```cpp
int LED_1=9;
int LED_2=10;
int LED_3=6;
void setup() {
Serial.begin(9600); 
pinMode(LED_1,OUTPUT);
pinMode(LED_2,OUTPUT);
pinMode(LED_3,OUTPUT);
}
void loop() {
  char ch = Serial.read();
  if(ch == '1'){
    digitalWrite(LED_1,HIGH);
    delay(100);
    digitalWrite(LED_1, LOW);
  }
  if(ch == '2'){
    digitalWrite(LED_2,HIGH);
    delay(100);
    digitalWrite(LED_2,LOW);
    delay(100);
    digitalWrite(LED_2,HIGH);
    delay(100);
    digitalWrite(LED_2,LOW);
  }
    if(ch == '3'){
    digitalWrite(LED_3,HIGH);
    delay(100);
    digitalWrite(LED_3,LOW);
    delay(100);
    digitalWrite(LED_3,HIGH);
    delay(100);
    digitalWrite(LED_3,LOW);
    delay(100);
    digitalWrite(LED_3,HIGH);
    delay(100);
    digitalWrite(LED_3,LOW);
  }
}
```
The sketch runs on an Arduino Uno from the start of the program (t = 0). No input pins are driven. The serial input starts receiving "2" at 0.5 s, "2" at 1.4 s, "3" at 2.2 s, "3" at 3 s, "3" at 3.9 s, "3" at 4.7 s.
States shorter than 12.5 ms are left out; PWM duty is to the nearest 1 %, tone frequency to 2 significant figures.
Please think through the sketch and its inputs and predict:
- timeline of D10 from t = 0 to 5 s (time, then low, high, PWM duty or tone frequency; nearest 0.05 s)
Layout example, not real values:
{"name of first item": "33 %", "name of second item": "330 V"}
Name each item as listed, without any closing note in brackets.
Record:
{"timeline of D10 from t = 0 to 5 s": "0 s low; 0.5 s high; 0.6 s low; 0.7 s high; 0.8 s low; 1.4 s high; 1.5 s low; 1.6 s high; 1.7 s low"}
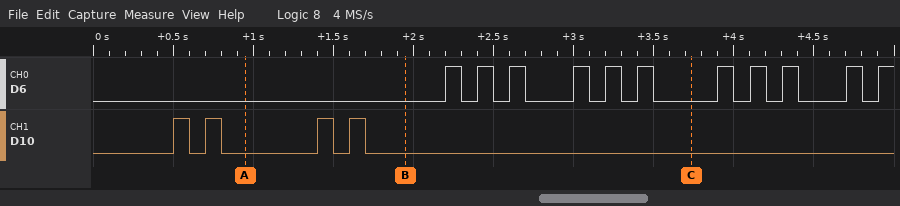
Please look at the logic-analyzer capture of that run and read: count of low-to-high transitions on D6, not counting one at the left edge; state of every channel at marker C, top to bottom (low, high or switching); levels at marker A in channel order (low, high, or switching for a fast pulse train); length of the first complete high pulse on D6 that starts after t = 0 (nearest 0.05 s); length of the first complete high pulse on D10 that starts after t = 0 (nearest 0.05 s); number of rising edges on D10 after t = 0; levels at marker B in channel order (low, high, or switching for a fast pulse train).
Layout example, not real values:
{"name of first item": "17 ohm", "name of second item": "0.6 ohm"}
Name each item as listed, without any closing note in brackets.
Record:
{"count of low-to-high transitions on D6, not counting one at the left edge": "11", "state of every channel at marker C, top to bottom": "D6 low, D10 low", "levels at marker A in channel order": "D6 low, D10 low", "length of the first complete high pulse on D6 that starts after t = 0": "0.10 s", "length of the first complete high pulse on D10 that starts after t = 0": "0.10 s", "number of rising edges on D10 after t = 0": "4", "levels at marker B in channel order": "D6 low, D10 low"}
